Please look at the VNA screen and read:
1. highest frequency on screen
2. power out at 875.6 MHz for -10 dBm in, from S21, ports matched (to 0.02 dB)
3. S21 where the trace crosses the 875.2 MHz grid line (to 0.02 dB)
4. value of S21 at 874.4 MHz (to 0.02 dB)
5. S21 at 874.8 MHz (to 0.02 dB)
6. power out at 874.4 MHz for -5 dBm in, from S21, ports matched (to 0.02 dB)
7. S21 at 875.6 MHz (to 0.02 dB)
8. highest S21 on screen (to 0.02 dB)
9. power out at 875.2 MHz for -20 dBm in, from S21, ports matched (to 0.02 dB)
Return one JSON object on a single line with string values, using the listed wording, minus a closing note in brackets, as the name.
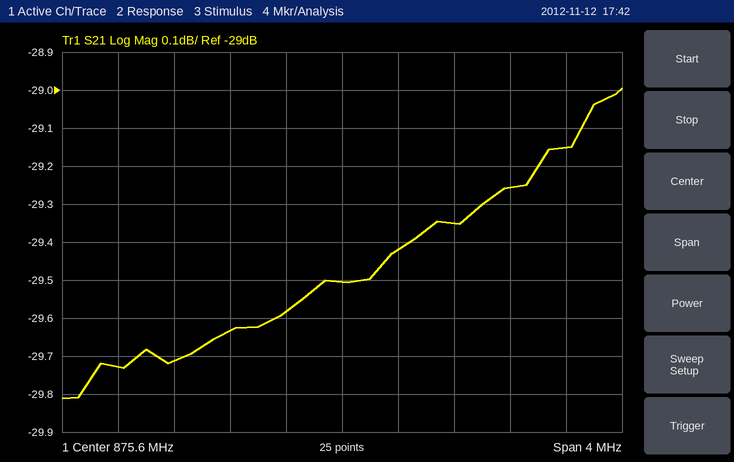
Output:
{"highest frequency on screen": "877.6 MHz", "power out at 875.6 MHz for -10 dBm in, from S21, ports matched": "-39.50 dBm", "S21 where the trace crosses the 875.2 MHz grid line": "-29.58 dB", "value of S21 at 874.4 MHz": "-29.72 dB", "S21 at 874.8 MHz": "-29.64 dB", "power out at 874.4 MHz for -5 dBm in, from S21, ports matched": "-34.72 dBm", "S21 at 875.6 MHz": "-29.50 dB", "highest S21 on screen": "-29.00 dB", "power out at 875.2 MHz for -20 dBm in, from S21, ports matched": "-49.58 dBm"}
